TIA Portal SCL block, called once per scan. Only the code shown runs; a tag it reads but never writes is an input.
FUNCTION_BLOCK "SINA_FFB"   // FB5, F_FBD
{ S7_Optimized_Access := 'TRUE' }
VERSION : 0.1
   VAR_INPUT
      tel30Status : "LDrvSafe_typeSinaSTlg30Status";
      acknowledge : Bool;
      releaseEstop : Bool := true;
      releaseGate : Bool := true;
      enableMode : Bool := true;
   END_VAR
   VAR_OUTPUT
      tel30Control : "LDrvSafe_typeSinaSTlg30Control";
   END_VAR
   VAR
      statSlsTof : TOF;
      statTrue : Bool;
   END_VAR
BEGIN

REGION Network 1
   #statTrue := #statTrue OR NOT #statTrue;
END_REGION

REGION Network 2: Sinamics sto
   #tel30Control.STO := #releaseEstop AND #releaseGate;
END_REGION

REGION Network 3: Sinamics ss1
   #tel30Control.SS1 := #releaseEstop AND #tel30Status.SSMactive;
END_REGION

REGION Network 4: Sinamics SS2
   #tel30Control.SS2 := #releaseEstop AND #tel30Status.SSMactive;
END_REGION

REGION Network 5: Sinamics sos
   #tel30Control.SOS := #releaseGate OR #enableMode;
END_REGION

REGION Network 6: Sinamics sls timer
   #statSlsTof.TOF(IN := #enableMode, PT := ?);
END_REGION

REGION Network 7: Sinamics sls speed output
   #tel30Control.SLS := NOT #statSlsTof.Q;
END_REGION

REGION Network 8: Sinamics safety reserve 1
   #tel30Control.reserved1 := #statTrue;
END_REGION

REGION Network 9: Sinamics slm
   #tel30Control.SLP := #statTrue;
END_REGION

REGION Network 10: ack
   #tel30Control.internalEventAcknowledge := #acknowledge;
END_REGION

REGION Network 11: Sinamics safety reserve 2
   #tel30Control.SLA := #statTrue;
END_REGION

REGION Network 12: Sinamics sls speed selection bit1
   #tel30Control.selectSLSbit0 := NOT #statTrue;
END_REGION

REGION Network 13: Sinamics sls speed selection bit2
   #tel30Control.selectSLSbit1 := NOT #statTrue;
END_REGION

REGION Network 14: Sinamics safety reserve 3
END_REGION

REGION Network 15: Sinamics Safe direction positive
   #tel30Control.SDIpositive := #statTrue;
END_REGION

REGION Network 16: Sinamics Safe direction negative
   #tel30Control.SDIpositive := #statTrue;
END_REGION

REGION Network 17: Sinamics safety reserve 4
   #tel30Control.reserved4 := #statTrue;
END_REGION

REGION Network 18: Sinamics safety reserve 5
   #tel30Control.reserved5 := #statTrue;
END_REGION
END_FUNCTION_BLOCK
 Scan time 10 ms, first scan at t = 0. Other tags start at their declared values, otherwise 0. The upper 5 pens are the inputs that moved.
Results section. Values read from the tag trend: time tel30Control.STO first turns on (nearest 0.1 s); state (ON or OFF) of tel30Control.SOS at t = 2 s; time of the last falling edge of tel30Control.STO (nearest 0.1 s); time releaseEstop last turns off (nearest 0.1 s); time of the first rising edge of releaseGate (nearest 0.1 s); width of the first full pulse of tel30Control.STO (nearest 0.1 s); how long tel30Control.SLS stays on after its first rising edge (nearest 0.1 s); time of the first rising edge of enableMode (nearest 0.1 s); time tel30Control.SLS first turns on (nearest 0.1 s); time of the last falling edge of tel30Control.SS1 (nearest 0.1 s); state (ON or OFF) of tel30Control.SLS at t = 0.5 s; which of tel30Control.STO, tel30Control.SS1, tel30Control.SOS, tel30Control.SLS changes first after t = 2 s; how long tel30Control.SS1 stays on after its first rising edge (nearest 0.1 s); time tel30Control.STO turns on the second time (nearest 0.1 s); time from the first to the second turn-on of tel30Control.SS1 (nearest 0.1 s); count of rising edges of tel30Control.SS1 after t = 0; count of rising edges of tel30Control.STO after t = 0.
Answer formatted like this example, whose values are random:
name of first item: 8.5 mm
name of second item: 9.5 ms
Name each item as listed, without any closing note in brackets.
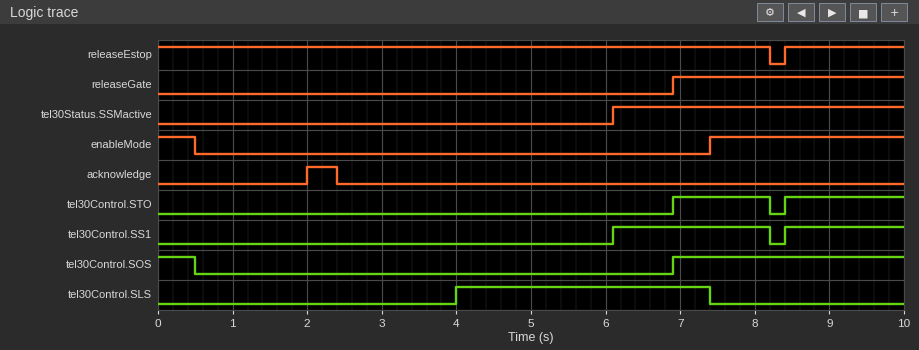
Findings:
time tel30Control.STO first turns on: 6.9 s
state (ON or OFF) of tel30Control.SOS at t = 2 s: OFF
time of the last falling edge of tel30Control.STO: 8.2 s
time releaseEstop last turns off: 8.2 s
time of the first rising edge of releaseGate: 6.9 s
width of the first full pulse of tel30Control.STO: 1.3 s
how long tel30Control.SLS stays on after its first rising edge: 3.4 s
time of the first rising edge of enableMode: 7.4 s
time tel30Control.SLS first turns on: 4.0 s
time of the last falling edge of tel30Control.SS1: 8.2 s
state (ON or OFF) of tel30Control.SLS at t = 0.5 s: OFF
which of tel30Control.STO, tel30Control.SS1, tel30Control.SOS, tel30Control.SLS changes first after t = 2 s: tel30Control.SLS
how long tel30Control.SS1 stays on after its first rising edge: 2.1 s
time tel30Control.STO turns on the second time: 8.4 s
time from the first to the second turn-on of tel30Control.SS1: 2.3 s
count of rising edges of tel30Control.SS1 after t = 0: 2
count of rising edges of tel30Control.STO after t = 0: 2
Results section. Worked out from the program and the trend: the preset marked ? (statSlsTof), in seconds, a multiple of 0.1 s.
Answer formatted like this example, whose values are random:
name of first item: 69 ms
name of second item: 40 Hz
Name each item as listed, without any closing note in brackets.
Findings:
the preset marked ? (statSlsTof), in seconds, a multiple of 0.1 s: 3.5 s
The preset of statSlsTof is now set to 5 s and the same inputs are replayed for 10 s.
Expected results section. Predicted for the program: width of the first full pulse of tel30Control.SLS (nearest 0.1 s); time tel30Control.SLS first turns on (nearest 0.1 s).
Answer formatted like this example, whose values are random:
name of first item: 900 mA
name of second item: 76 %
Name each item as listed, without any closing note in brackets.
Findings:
width of the first full pulse of tel30Control.SLS: 1.9 s
time tel30Control.SLS first turns on: 5.5 s
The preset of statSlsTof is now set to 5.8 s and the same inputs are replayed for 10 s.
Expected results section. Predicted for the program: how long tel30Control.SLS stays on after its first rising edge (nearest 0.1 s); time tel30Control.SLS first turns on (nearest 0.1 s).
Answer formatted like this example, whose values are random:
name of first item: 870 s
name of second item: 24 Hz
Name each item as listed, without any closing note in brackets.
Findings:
how long tel30Control.SLS stays on after its first rising edge: 1.1 s
time tel30Control.SLS first turns on: 6.3 s
